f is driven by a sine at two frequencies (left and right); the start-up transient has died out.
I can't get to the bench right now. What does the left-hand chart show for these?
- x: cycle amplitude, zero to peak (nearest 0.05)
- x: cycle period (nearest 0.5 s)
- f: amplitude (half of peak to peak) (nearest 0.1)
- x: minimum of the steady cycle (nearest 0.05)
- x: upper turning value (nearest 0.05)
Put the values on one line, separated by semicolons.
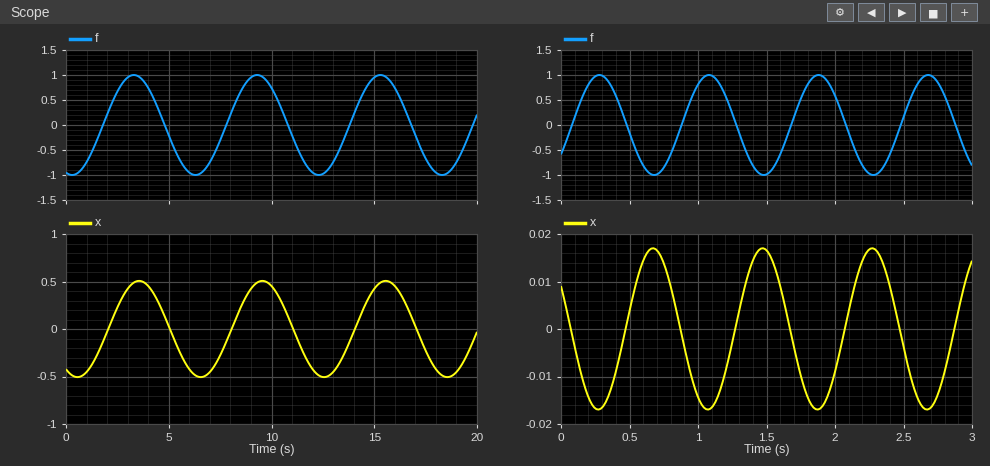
0.50; 6.0 s; 1.0; -0.50; 0.50
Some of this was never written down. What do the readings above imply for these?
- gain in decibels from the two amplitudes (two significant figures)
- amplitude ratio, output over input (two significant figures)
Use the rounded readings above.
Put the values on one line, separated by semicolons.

-6.0 dB; 0.50
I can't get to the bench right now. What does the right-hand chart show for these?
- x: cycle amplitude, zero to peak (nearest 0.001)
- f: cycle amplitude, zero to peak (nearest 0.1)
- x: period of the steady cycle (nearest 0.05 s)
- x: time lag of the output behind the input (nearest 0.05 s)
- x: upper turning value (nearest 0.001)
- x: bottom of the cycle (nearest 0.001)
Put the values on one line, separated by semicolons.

0.017; 1.0; 0.80 s; 0.40 s; 0.017; -0.017
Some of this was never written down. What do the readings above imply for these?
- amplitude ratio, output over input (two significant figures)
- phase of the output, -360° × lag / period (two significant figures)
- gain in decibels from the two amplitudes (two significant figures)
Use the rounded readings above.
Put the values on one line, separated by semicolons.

0.017; -180°; -35 dB
